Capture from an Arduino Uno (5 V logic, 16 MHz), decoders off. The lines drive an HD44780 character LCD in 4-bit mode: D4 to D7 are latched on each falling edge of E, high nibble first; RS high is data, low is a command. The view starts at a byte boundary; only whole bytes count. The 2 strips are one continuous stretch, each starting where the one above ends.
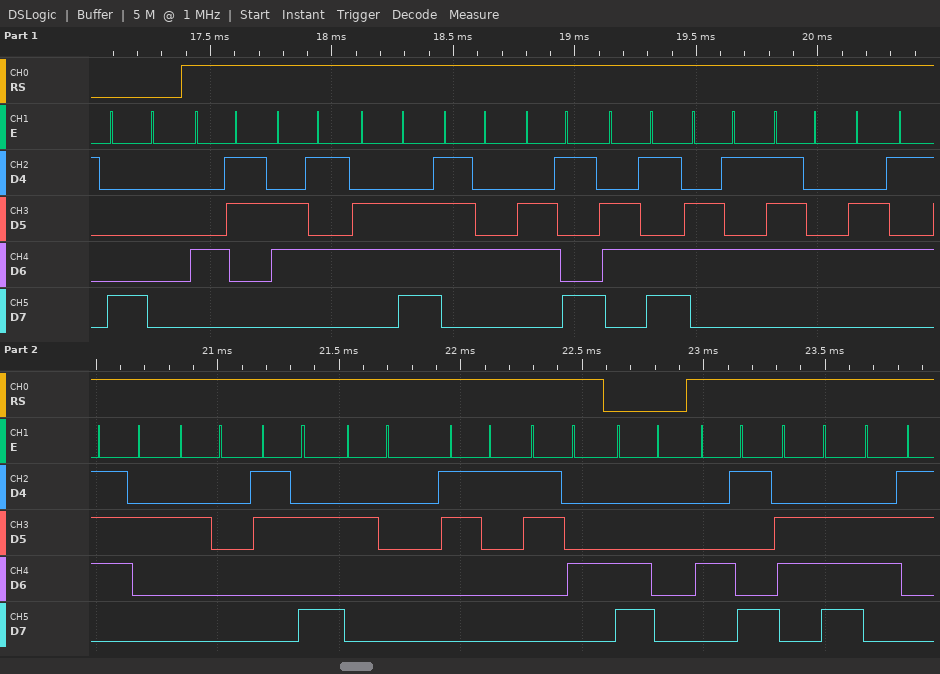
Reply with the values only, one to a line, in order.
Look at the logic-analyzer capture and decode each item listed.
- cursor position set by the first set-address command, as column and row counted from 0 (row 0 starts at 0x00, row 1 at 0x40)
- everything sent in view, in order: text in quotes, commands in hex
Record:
column 0, row 0
0x80 "Centimeter : 14" 0xC0 "Inc"
